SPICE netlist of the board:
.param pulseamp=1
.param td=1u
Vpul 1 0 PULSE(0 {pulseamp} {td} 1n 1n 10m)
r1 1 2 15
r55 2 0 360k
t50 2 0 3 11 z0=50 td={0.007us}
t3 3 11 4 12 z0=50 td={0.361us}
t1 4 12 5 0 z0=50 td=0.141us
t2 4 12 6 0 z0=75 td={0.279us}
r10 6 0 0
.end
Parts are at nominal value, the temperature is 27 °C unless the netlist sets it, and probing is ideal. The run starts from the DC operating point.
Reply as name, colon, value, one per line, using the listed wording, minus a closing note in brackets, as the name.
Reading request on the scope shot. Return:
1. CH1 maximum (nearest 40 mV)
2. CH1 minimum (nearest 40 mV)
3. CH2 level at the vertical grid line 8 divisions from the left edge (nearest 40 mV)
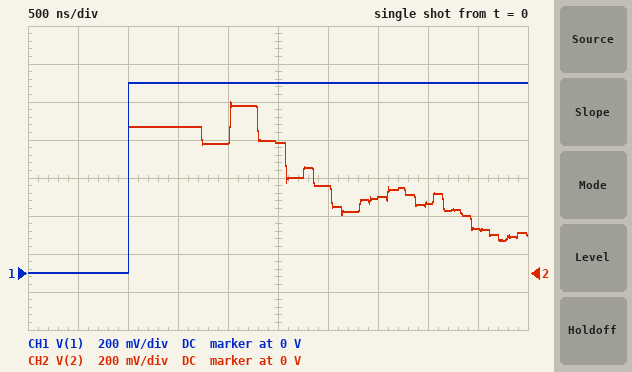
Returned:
CH1 maximum: 1.00 V
CH1 minimum: 0 V
CH2 level at the vertical grid line 8 divisions from the left edge: 360 mV
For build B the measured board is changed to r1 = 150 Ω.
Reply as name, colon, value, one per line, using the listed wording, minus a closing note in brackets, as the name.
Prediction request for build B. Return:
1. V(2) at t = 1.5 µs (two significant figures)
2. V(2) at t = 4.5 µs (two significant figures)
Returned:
V(2) at t = 1.5 µs: 250 mV
V(2) at t = 4.5 µs: 50 mV
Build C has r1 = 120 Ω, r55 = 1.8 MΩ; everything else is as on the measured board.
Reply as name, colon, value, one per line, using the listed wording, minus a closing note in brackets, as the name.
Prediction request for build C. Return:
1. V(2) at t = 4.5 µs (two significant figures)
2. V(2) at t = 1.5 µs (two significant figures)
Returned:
V(2) at t = 4.5 µs: 39 mV
V(2) at t = 1.5 µs: 290 mV
